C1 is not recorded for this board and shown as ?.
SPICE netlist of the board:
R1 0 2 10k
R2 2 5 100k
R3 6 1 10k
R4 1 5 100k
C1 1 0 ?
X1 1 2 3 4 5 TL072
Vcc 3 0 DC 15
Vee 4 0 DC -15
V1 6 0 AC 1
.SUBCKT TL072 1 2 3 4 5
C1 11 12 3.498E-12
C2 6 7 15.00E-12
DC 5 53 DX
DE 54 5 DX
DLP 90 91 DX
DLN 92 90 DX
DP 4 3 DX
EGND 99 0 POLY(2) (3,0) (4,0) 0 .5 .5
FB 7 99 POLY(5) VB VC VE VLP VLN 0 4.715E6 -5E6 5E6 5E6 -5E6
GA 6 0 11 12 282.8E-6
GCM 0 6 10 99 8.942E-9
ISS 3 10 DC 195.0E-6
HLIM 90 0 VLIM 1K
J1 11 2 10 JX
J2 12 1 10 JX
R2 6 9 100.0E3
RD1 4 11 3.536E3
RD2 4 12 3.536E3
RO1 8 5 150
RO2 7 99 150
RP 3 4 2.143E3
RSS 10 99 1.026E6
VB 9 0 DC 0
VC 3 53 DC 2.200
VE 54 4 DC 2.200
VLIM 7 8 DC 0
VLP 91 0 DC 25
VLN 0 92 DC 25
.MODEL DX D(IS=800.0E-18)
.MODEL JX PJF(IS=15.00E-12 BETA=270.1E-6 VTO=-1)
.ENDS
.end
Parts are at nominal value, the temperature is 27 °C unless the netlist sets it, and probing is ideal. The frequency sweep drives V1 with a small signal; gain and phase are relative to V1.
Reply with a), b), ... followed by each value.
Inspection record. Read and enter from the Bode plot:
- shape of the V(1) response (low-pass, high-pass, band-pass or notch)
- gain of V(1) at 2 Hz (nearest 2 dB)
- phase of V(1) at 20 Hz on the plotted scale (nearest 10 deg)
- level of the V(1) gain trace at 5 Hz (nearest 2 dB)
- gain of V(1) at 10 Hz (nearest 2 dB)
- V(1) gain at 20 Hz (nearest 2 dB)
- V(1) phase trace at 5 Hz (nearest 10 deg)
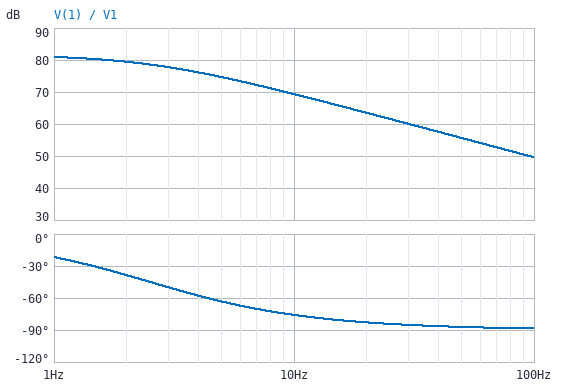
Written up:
a) low-pass
b) 80 dB
c) -80 deg
d) 74 dB
e) 70 dB
f) 64 dB
g) -60 deg
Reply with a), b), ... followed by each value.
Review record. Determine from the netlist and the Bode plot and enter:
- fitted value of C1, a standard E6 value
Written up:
a) 470 pF
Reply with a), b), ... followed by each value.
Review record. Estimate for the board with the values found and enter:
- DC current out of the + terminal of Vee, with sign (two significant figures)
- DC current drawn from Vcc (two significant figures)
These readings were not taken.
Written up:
a) -14 mA
b) 14 mA
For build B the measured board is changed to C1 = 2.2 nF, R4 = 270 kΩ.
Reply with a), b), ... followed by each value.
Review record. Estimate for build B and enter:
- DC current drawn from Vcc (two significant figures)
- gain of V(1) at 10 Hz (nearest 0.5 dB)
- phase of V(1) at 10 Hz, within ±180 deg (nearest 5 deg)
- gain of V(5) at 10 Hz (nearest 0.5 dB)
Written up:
a) 14 mA
b) 4.0 dB
c) 0 deg
d) 25.0 dB
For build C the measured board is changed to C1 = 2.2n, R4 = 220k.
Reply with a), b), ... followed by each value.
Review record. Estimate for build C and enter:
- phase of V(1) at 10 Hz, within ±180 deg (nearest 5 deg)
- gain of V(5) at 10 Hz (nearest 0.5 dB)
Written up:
a) 0 deg
b) 26.0 dB
